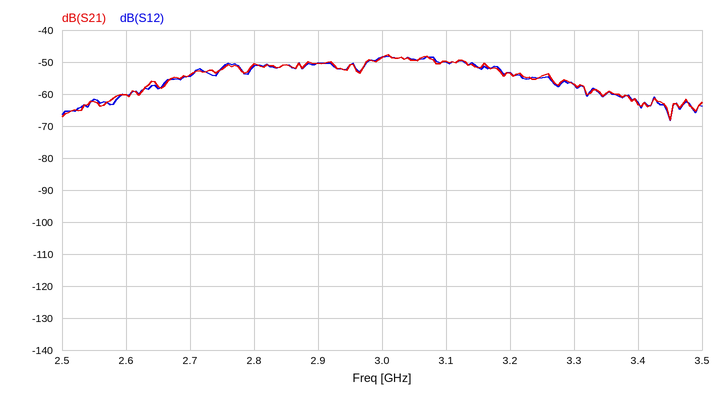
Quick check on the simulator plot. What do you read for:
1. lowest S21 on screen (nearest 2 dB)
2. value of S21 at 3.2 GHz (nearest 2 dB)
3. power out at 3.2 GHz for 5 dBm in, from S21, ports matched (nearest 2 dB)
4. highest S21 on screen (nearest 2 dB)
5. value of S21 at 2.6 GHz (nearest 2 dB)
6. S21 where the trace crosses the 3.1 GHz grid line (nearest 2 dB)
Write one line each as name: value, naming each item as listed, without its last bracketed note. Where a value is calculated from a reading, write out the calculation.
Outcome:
lowest S21 on screen: -68 dB
value of S21 at 3.2 GHz: -54 dB
power out at 3.2 GHz for 5 dBm in, from S21, ports matched: 5 dBm + (-54 dB) = -48 dBm
highest S21 on screen: -48 dB
value of S21 at 2.6 GHz: -60 dB
S21 where the trace crosses the 3.1 GHz grid line: -50 dB
